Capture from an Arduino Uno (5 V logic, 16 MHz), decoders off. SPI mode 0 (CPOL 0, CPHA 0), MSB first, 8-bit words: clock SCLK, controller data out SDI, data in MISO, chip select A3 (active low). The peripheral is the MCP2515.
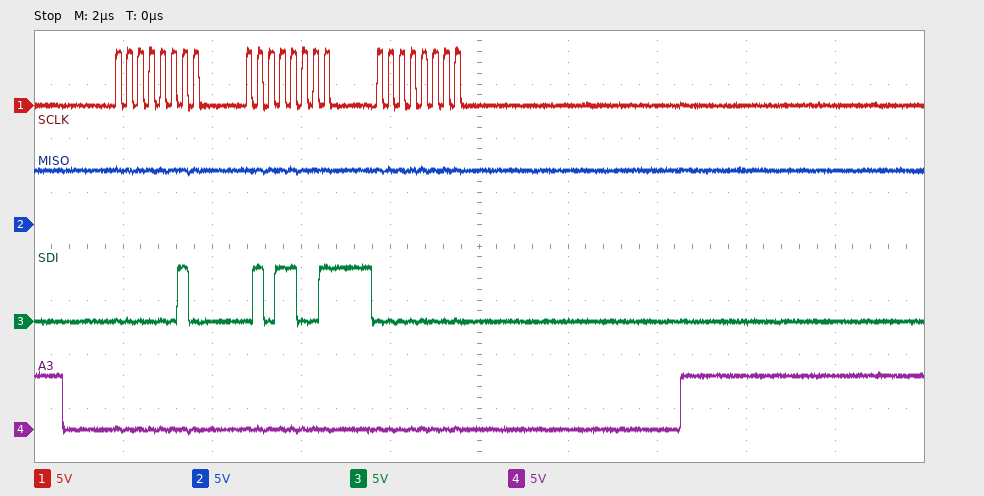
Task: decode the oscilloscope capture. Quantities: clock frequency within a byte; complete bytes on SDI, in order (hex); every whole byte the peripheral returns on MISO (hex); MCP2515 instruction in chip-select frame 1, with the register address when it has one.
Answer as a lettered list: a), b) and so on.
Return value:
a) 4 MHz
b) 02 59 00
c) FF FF FF
d) WRITE 0x59
